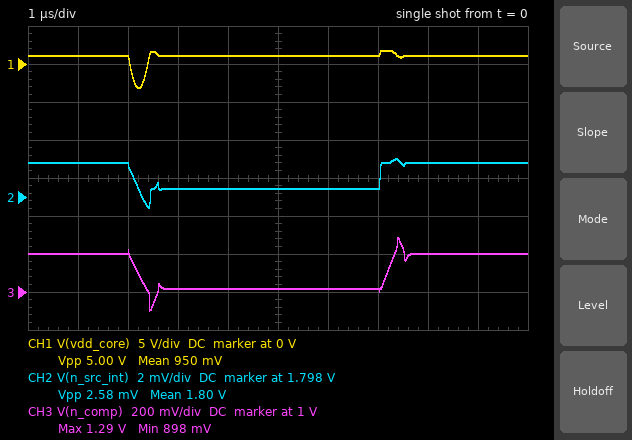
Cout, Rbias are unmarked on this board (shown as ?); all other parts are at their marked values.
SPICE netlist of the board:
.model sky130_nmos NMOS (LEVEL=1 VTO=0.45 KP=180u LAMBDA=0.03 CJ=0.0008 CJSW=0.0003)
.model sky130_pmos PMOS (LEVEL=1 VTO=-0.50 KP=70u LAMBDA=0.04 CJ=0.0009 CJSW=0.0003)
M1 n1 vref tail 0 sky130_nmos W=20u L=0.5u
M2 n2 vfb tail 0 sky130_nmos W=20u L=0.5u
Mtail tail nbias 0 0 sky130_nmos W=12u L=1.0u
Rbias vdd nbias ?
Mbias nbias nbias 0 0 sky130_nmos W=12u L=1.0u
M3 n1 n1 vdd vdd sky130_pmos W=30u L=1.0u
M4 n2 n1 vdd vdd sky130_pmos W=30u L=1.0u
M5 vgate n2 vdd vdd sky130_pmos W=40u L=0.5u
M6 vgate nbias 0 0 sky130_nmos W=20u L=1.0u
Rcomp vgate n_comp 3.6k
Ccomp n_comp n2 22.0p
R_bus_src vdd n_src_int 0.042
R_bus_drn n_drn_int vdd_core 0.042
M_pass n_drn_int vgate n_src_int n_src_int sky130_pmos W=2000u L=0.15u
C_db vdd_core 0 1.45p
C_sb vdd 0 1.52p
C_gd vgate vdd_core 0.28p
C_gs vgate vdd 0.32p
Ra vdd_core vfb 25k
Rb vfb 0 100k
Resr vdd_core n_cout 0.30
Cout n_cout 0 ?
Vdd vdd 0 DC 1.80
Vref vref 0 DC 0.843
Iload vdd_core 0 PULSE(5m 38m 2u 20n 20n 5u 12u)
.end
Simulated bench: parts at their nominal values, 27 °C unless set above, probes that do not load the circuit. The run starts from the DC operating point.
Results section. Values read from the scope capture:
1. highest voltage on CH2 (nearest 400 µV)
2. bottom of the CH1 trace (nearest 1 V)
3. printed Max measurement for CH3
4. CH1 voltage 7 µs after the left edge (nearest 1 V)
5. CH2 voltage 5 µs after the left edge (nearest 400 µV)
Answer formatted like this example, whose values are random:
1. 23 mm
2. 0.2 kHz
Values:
1. 1.8000 V
2. -3 V
3. 1.29 V
4. 1 V
5. 1.7984 V
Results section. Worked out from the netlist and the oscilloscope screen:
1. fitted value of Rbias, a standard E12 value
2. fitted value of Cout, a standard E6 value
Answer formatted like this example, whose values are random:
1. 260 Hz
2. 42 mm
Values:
1. 82 kΩ
2. 680 pF
